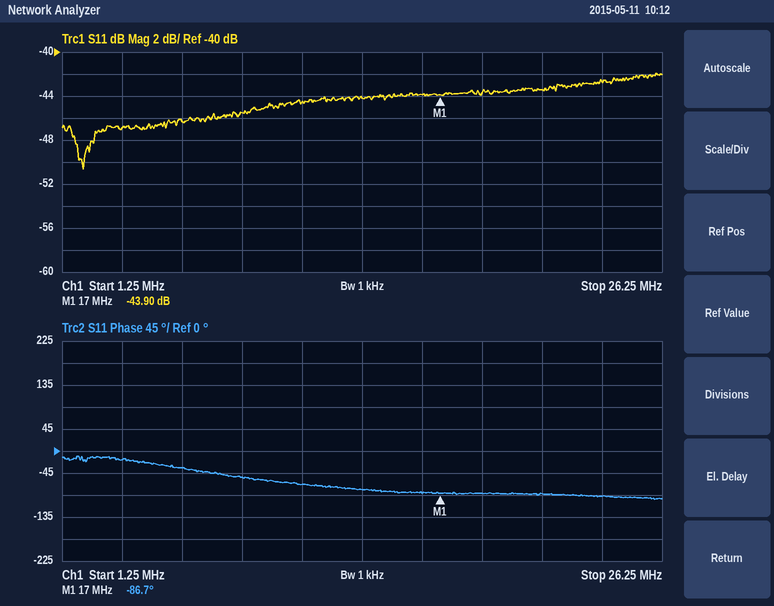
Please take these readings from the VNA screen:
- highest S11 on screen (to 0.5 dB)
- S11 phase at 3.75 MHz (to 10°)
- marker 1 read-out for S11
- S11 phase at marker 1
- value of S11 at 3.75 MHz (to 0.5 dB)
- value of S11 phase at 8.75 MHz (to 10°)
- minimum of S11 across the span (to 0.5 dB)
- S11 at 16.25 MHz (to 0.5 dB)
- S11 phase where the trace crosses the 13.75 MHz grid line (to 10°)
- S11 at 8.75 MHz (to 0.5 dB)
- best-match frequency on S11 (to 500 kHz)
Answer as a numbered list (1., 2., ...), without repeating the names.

1. -42.0 dB
2. -20°
3. -43.90 dB
4. -86.7°
5. -47.0 dB
6. -50°
7. -50.5 dB
8. -44.0 dB
9. -80°
10. -45.5 dB
11. 2.0 MHz
